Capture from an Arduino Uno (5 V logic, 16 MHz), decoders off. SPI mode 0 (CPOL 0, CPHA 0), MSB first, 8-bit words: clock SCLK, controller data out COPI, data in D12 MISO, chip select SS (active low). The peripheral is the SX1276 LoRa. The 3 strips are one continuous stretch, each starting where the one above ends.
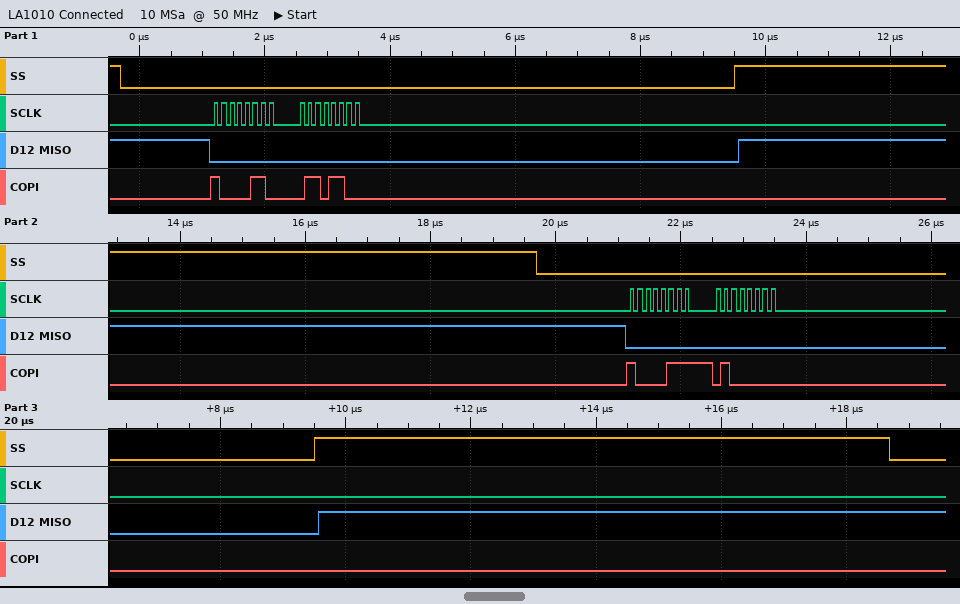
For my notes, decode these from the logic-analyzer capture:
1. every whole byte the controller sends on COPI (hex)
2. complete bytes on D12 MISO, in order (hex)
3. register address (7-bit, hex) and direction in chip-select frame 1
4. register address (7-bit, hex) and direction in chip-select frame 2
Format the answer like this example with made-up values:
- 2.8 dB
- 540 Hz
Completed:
- 86 6C 87 40
- 00 00 00 00
- 0x06 write
- 0x07 write
